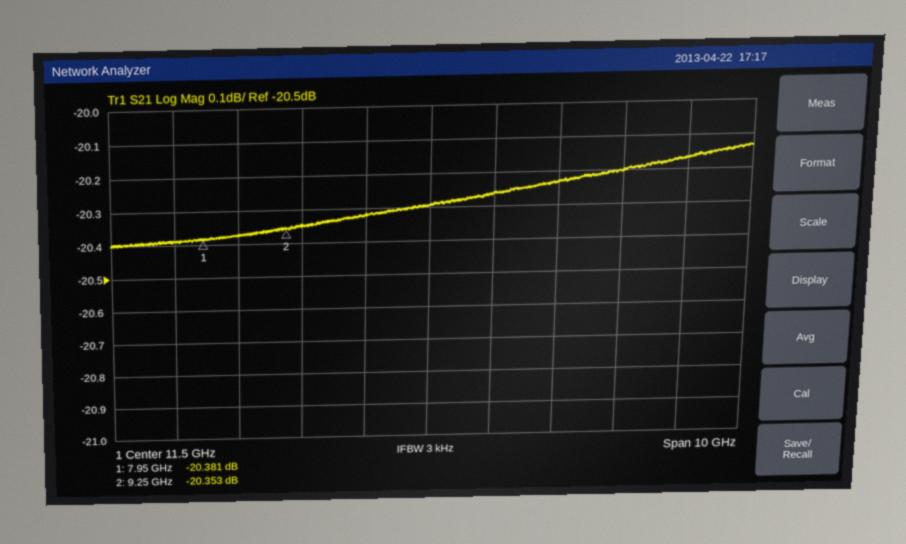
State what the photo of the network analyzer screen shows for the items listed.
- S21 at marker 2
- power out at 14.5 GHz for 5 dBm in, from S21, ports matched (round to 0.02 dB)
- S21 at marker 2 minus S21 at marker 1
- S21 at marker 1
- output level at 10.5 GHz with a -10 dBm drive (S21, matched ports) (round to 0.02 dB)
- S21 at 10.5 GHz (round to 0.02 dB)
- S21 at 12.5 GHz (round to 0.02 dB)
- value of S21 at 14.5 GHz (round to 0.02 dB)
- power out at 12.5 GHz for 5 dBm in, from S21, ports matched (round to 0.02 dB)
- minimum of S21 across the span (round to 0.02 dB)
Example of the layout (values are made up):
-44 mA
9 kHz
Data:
-20.353 dB
-15.20 dBm
0.028 dB
-20.381 dB
-30.32 dBm
-20.32 dB
-20.26 dB
-20.20 dB
-15.26 dBm
-20.40 dB
